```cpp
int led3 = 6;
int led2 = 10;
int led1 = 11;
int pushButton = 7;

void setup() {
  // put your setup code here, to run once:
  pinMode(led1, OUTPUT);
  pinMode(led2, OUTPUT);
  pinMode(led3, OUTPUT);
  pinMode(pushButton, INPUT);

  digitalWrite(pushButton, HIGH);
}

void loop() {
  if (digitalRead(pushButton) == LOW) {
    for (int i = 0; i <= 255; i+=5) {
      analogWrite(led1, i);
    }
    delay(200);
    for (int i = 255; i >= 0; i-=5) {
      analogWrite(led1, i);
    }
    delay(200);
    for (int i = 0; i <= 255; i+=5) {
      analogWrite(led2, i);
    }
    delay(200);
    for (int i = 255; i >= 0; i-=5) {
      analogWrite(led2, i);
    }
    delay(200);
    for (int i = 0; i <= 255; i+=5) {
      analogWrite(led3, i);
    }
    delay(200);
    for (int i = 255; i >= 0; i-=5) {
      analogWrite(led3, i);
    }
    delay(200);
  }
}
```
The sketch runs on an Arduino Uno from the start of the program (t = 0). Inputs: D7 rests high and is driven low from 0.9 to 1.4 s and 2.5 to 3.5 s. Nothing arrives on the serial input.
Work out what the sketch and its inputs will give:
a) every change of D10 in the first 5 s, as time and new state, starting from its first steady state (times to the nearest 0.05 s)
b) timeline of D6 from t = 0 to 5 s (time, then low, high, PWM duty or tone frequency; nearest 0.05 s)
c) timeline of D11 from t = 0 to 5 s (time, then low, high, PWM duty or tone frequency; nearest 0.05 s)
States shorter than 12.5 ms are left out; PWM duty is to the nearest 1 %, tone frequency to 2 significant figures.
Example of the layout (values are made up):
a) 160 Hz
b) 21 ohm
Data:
a) 0 s low; 1.3 s high; 1.5 s low; 2.9 s high; 3.1 s low
b) 0 s low; 1.7 s high; 1.9 s low; 3.3 s high; 3.5 s low
c) 0 s low; 0.9 s high; 1.1 s low; 2.5 s high; 2.7 s low
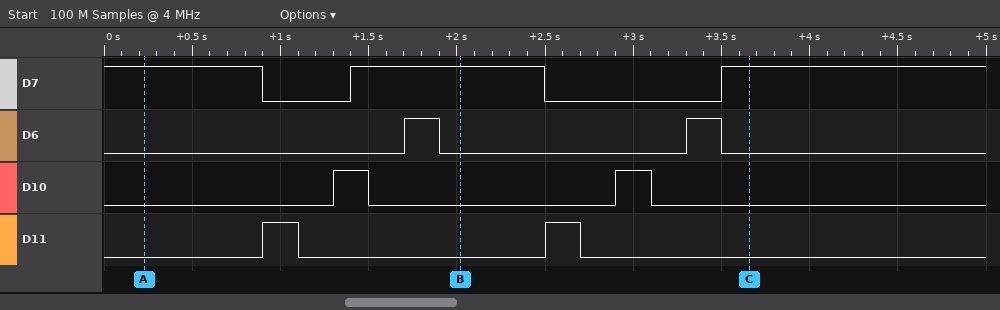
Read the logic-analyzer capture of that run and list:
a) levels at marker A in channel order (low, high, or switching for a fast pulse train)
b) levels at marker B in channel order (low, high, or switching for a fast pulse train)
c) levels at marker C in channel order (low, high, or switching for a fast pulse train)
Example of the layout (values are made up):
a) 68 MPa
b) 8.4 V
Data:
a) D7 high, D6 low, D10 low, D11 low
b) D7 high, D6 low, D10 low, D11 low
c) D7 high, D6 low, D10 low, D11 low
